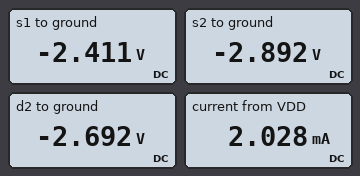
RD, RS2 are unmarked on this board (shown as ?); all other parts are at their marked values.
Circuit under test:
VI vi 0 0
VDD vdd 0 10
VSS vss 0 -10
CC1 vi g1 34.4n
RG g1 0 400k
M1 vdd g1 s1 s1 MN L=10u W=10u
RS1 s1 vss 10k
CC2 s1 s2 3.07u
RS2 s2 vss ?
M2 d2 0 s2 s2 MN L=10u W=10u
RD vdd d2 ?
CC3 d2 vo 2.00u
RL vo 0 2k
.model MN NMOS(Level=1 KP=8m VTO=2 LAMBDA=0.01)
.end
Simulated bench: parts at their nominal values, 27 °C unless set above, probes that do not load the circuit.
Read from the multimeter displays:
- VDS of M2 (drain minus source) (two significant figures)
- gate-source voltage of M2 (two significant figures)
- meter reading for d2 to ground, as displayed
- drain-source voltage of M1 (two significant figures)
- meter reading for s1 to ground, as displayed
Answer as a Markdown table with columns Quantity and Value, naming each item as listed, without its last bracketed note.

| Quantity | Value |
|---|---|
| VDS of M2 (drain minus source) | 200 mV |
| gate-source voltage of M2 | 2.9 V |
| meter reading for d2 to ground, as displayed | -2.692 V |
| drain-source voltage of M1 | 12 V |
| meter reading for s1 to ground, as displayed | -2.411 V |
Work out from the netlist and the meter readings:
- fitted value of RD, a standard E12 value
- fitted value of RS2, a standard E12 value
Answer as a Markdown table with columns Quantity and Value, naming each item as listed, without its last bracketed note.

| Quantity | Value |
|---|---|
| fitted value of RD, a standard E12 value | 10 kΩ |
| fitted value of RS2, a standard E12 value | 5.6 kΩ |
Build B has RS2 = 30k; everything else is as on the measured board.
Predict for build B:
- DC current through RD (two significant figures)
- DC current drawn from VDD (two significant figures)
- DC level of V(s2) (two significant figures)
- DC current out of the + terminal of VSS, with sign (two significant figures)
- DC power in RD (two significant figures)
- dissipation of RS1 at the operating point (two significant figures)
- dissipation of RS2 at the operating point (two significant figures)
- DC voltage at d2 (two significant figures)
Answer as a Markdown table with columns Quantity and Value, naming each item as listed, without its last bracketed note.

| Quantity | Value |
|---|---|
| DC current through RD | 260 µA |
| DC current drawn from VDD | 1.0 mA |
| DC level of V(s2) | -2.2 V |
| DC current out of the + terminal of VSS, with sign | -1.0 mA |
| DC power in RD | 670 µW |
| dissipation of RS1 at the operating point | 5.8 mW |
| dissipation of RS2 at the operating point | 2.0 mW |
| DC voltage at d2 | 7.4 V |
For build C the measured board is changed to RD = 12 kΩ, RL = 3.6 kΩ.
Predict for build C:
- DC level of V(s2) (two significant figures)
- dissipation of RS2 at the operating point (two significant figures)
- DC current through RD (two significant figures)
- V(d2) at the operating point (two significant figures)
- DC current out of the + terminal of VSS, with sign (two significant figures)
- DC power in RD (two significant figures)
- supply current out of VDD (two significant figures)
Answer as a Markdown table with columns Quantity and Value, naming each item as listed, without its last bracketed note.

| Quantity | Value |
|---|---|
| DC level of V(s2) | -3.7 V |
| dissipation of RS2 at the operating point | 7.2 mW |
| DC current through RD | 1.1 mA |
| V(d2) at the operating point | -3.6 V |
| DC current out of the + terminal of VSS, with sign | -1.9 mA |
| DC power in RD | 15 mW |
| supply current out of VDD | 1.9 mA |
